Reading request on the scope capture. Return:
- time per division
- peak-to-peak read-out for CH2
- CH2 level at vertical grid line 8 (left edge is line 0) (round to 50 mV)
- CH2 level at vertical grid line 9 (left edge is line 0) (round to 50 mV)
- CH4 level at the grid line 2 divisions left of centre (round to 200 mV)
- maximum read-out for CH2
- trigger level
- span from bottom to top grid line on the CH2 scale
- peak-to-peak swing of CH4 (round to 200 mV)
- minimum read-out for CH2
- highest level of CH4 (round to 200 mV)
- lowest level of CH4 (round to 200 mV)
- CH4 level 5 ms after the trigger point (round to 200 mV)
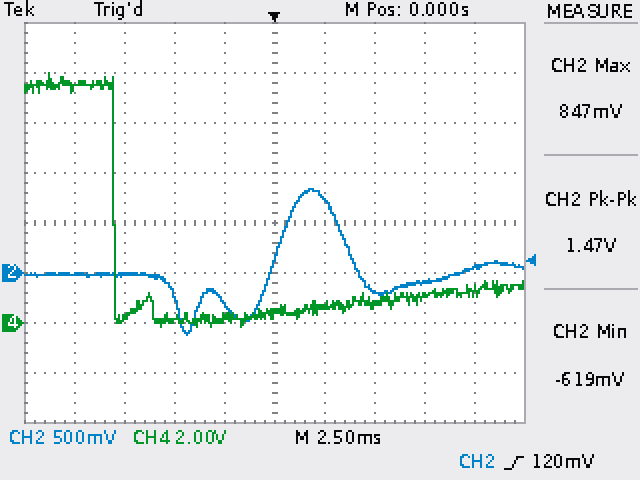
2.5 ms
1.47 V
-100 mV
50 mV
200 mV
847 mV
120 mV
4 V
10.2 V
-619 mV
10.0 V
-200 mV
800 mV
